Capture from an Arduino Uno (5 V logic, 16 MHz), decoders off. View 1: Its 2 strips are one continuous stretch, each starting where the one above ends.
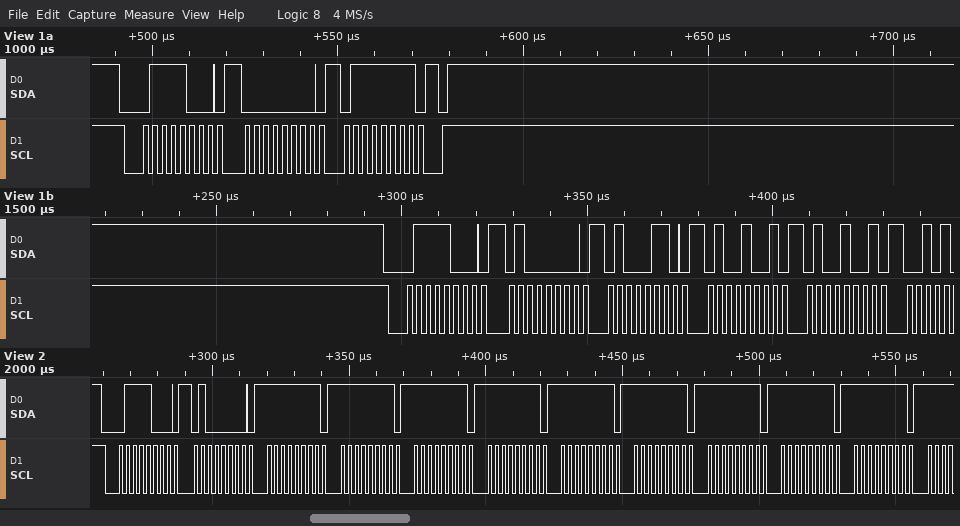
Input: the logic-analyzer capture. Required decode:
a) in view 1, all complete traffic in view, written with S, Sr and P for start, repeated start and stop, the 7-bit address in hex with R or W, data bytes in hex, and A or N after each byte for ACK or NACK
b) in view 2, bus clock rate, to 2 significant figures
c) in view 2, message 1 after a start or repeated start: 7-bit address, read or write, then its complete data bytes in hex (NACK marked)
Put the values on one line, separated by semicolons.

S 3CW A 00 A 7F A P S 3CW A 40 A 46 A 49 A 49 A; 400 kHz; 0x3C write: 40 FF FF FF FF FF FF FF FF FF
